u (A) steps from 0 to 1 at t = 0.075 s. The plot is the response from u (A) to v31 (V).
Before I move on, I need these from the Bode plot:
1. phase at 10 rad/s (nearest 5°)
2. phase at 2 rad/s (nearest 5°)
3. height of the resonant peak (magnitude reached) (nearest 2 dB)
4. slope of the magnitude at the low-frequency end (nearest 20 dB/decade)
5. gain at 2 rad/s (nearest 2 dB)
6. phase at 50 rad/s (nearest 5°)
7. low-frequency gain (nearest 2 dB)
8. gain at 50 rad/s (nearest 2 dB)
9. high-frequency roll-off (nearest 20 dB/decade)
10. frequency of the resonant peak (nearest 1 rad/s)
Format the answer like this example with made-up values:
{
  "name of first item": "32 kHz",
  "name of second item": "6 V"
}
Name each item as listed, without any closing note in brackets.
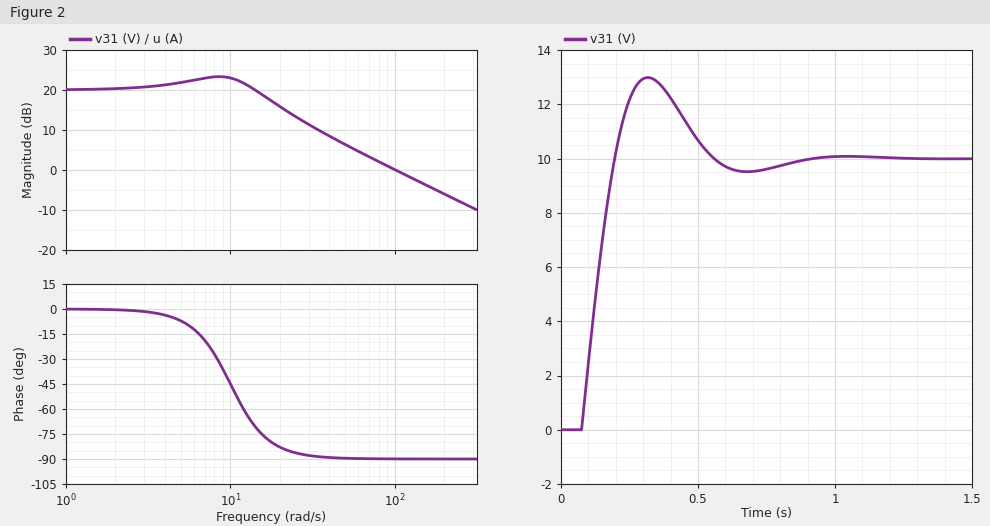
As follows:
{
  "phase at 10 rad/s": "-45°",
  "phase at 2 rad/s": "0°",
  "height of the resonant peak (magnitude reached)": "24 dB",
  "slope of the magnitude at the low-frequency end": "0 dB/decade",
  "gain at 2 rad/s": "20 dB",
  "phase at 50 rad/s": "-90°",
  "low-frequency gain": "20 dB",
  "gain at 50 rad/s": "6 dB",
  "high-frequency roll-off": "-20 dB/decade",
  "frequency of the resonant peak": "8 rad/s"
}
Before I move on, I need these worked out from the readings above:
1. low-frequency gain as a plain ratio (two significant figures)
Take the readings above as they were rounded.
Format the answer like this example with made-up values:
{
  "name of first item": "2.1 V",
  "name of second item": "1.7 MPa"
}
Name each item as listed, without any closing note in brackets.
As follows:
{
  "low-frequency gain as a plain ratio": "10"
}
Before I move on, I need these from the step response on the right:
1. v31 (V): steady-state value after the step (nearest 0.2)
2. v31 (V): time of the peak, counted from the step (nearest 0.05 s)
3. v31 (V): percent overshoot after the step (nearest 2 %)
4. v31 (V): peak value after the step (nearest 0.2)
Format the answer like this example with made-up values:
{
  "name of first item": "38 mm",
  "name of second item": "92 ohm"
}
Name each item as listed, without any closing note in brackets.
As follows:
{
  "v31 (V): steady-state value after the step": "10.0",
  "v31 (V): time of the peak, counted from the step": "0.25 s",
  "v31 (V): percent overshoot after the step": "30 %",
  "v31 (V): peak value after the step": "13.0"
}
